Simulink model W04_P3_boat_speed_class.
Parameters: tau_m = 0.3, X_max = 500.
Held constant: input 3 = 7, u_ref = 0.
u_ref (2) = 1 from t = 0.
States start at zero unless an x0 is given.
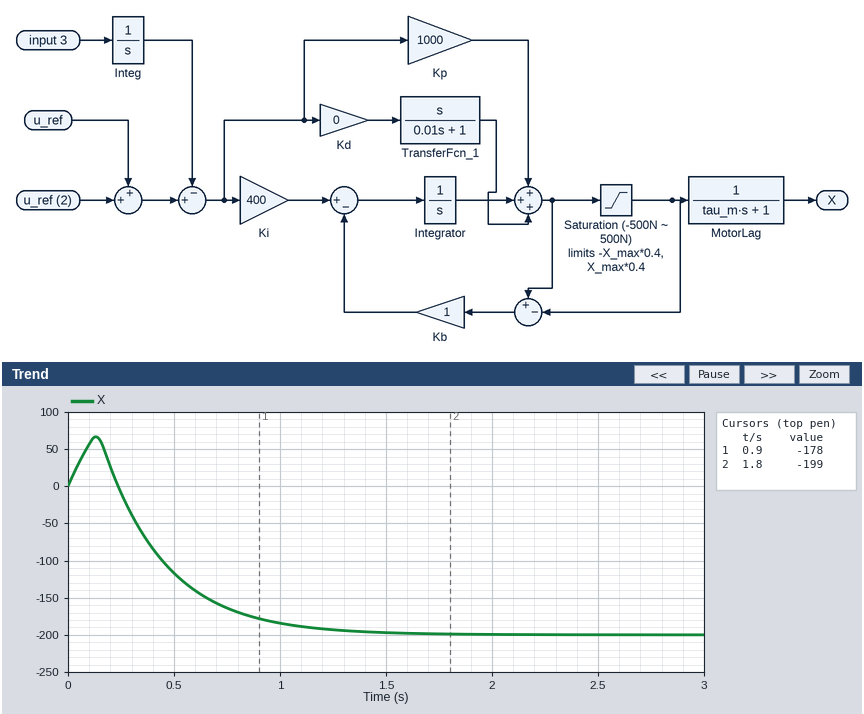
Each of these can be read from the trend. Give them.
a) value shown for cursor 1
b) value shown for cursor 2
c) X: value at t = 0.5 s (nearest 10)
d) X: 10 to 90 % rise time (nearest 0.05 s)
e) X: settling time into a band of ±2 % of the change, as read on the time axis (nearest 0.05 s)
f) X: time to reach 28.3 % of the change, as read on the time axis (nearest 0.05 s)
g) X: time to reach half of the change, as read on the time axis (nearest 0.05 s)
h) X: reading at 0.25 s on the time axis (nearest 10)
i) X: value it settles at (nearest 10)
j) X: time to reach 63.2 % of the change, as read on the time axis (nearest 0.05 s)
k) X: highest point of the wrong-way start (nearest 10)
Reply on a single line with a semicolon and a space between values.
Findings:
-178; -199; -120; 0.65 s; 1.40 s; 0.35 s; 0.45 s; -10; -200; 0.55 s; 70
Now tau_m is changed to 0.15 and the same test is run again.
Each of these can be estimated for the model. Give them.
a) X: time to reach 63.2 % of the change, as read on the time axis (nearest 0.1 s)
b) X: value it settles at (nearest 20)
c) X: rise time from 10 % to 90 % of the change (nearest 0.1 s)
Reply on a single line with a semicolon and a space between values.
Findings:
0.4 s; -200; 0.3 s
